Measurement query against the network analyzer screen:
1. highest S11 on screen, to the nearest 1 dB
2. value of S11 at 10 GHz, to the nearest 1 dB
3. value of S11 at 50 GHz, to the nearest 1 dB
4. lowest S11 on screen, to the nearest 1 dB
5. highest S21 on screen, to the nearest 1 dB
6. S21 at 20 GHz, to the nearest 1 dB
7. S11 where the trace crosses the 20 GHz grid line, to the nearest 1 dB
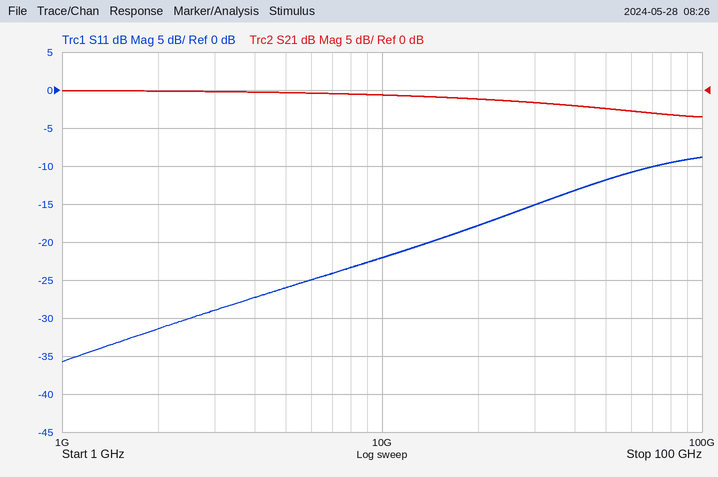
-9 dB
-22 dB
-12 dB
-36 dB
0 dB
-1 dB
-18 dB
